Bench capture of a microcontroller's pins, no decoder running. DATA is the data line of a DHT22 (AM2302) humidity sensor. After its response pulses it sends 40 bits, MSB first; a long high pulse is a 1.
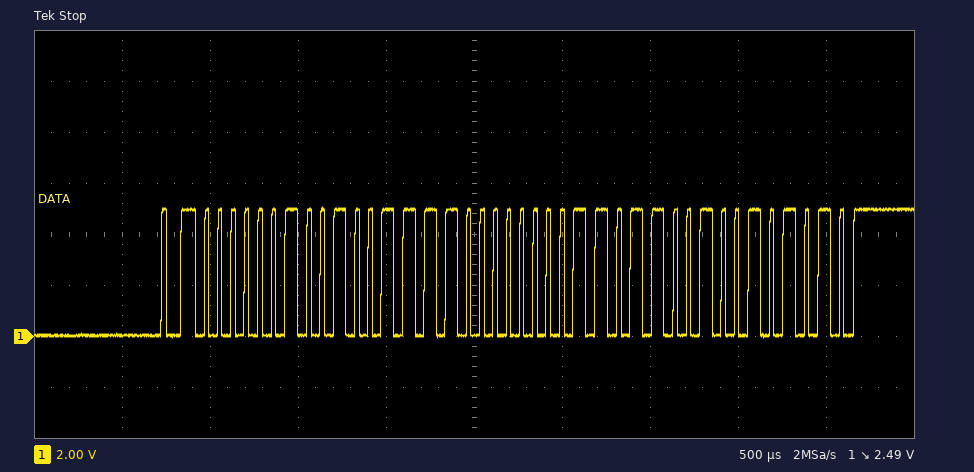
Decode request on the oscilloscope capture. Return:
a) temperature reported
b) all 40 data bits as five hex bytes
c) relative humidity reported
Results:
21.7 °C
02 4F 00 D9 2A
59.1 %
